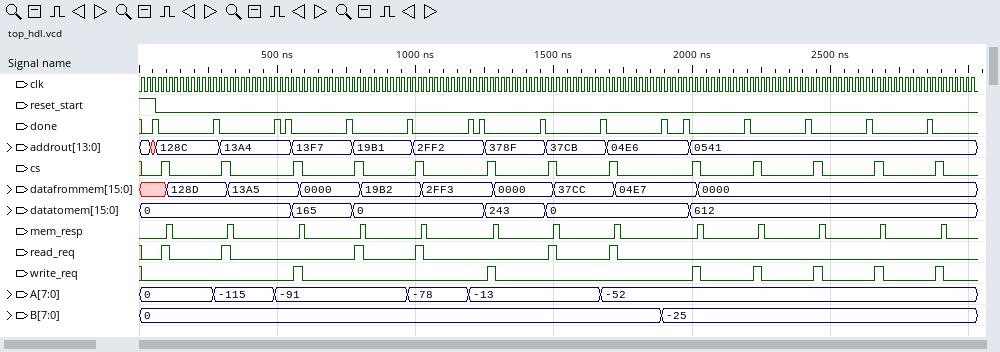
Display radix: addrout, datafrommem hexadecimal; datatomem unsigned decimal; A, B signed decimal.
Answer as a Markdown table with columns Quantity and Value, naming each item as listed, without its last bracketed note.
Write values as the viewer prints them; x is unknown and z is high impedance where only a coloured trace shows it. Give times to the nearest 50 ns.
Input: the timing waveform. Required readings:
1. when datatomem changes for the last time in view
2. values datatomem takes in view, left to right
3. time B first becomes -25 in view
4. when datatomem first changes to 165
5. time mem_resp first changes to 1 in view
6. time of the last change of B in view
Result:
| Quantity | Value |
|---|---|
| when datatomem changes for the last time in view | 2000 ns |
| values datatomem takes in view, left to right | 0, 165, 0, 243, 0, 612 |
| time B first becomes -25 in view | 1900 ns |
| when datatomem first changes to 165 | 550 ns |
| time mem_resp first changes to 1 in view | 100 ns |
| time of the last change of B in view | 1900 ns |
